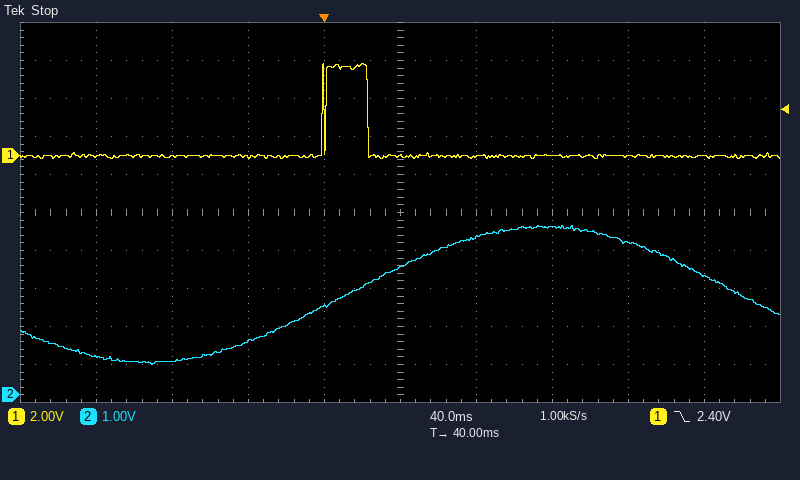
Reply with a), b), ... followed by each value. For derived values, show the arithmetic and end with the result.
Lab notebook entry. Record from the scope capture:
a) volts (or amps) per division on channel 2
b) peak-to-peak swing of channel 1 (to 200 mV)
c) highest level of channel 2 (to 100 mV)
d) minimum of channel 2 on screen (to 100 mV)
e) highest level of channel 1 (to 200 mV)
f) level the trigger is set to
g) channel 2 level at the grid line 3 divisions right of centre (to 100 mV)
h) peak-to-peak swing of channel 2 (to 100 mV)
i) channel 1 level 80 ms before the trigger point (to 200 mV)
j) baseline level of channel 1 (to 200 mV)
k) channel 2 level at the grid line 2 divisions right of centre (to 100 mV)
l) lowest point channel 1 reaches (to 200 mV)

a) 1 V
b) 4.8 V − (-200 mV) = 5.0 V
c) 4.5 V
d) 800 mV
e) 4.8 V
f) 2.40 V
g) 4.0 V
h) 4.5 V − (800 mV) = 3.7 V
i) 0.0 V
j) 0.0 V
k) 4.4 V
l) -200 mV
